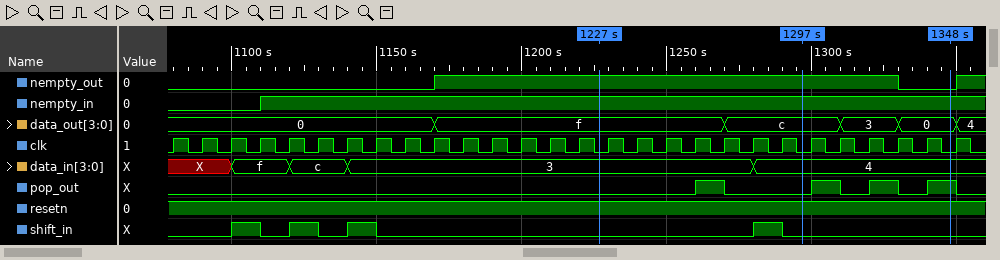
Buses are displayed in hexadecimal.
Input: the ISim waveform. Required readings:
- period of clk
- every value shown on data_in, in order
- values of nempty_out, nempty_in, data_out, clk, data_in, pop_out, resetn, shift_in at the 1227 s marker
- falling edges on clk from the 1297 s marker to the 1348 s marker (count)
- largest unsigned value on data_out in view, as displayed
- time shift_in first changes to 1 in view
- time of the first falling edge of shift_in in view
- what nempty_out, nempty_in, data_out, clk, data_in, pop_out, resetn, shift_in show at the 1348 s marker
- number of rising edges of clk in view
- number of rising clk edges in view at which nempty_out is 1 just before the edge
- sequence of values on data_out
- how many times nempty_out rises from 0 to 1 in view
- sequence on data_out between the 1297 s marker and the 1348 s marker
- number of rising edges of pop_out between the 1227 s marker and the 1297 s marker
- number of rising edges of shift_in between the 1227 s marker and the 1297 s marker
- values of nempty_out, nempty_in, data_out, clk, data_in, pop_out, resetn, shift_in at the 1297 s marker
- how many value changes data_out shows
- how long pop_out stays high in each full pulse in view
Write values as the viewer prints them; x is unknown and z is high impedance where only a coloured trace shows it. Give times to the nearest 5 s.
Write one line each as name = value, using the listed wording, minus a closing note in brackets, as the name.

period of clk = 10 s
every value shown on data_in, in order = X, f, c, 3, 4
values of nempty_out, nempty_in, data_out, clk, data_in, pop_out, resetn, shift_in at the 1227 s marker = nempty_out=1, nempty_in=1, data_out=f, clk=0, data_in=3, pop_out=0, resetn=1, shift_in=0
falling edges on clk from the 1297 s marker to the 1348 s marker = 5
largest unsigned value on data_out in view, as displayed = f
time shift_in first changes to 1 in view = 1100 s
time of the first falling edge of shift_in in view = 1110 s
what nempty_out, nempty_in, data_out, clk, data_in, pop_out, resetn, shift_in show at the 1348 s marker = nempty_out=0, nempty_in=1, data_out=0, clk=0, data_in=4, pop_out=1, resetn=1, shift_in=0
number of rising edges of clk in view = 28
number of rising clk edges in view at which nempty_out is 1 just before the edge = 16
sequence of values on data_out = 0, f, c, 3, 0, 4
how many times nempty_out rises from 0 to 1 in view = 2
sequence on data_out between the 1297 s marker and the 1348 s marker = c, 3, 0
number of rising edges of pop_out between the 1227 s marker and the 1297 s marker = 1
number of rising edges of shift_in between the 1227 s marker and the 1297 s marker = 1
values of nempty_out, nempty_in, data_out, clk, data_in, pop_out, resetn, shift_in at the 1297 s marker = nempty_out=1, nempty_in=1, data_out=c, clk=0, data_in=4, pop_out=0, resetn=1, shift_in=0
how many value changes data_out shows = 5
how long pop_out stays high in each full pulse in view = 10 s, 10 s, 10 s, 10 s
